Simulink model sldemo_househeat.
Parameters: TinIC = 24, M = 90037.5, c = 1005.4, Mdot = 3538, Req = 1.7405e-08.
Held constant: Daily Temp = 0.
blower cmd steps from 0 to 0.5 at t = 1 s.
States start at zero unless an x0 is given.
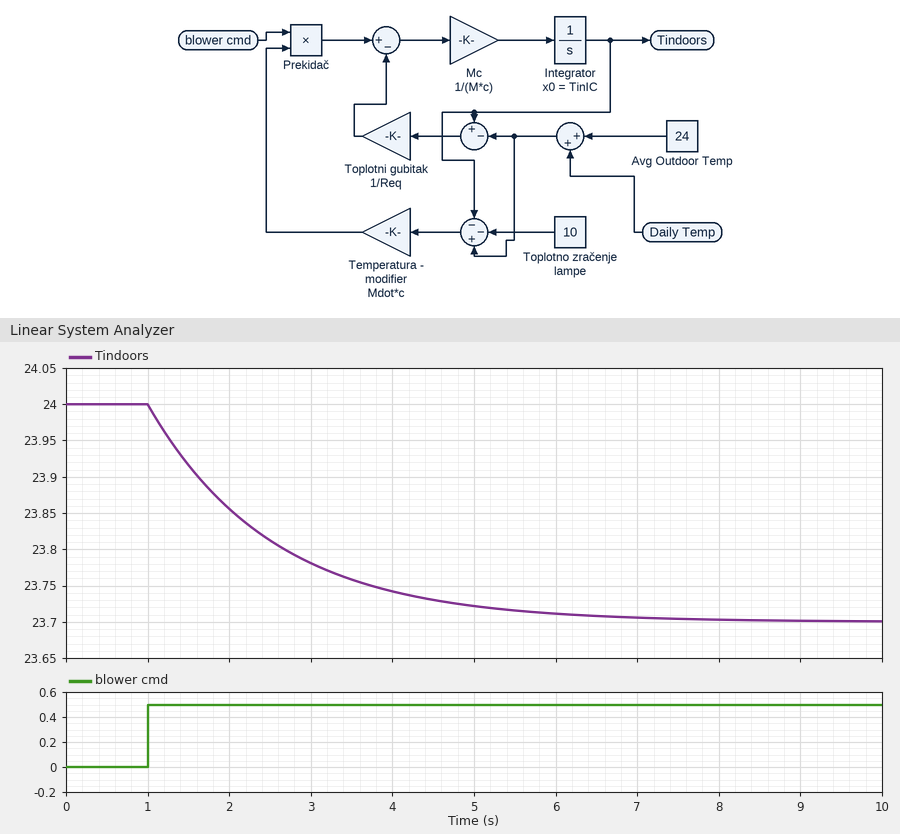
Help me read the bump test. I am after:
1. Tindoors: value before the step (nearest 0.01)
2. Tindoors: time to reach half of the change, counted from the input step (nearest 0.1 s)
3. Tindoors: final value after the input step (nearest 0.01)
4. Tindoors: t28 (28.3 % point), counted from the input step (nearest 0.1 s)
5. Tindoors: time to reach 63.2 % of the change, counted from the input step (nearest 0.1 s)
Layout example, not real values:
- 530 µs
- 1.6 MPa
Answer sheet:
- 24.00
- 1.1 s
- 23.70
- 0.5 s
- 1.5 s
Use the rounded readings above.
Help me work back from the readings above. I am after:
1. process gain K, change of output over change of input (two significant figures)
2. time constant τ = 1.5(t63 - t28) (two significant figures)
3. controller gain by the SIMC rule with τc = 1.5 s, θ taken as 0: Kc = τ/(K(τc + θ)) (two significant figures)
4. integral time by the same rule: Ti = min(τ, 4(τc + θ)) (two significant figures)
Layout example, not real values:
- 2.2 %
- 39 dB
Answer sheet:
- -0.60
- 1.5 s
- -1.7
- 1.5 s
